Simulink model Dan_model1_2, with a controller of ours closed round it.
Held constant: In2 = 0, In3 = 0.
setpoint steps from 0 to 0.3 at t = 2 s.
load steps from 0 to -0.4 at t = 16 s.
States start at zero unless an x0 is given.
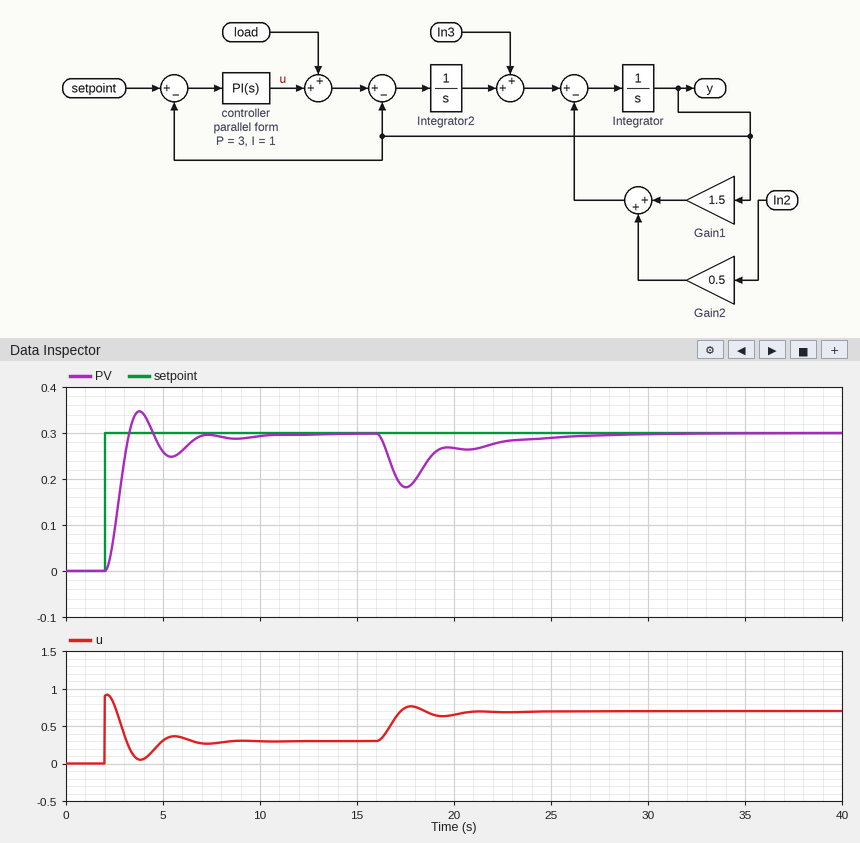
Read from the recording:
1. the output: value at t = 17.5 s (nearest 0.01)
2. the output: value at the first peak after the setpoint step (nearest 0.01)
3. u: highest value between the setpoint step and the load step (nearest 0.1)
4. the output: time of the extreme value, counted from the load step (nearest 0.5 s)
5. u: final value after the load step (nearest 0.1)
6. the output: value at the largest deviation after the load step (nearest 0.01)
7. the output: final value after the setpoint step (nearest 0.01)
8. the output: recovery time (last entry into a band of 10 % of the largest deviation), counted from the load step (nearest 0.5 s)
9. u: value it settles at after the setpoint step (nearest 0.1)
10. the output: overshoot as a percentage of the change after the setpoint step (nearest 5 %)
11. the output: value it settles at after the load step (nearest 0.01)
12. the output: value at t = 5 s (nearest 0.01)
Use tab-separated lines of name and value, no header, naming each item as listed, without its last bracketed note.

the output: value at t = 17.5 s	0.18
the output: value at the first peak after the setpoint step	0.35
u: highest value between the setpoint step and the load step	0.9
the output: time of the extreme value, counted from the load step	1.5 s
u: final value after the load step	0.7
the output: value at the largest deviation after the load step	0.18
the output: final value after the setpoint step	0.30
the output: recovery time (last entry into a band of 10 % of the largest deviation), counted from the load step	8.5 s
u: value it settles at after the setpoint step	0.3
the output: overshoot as a percentage of the change after the setpoint step	15 %
the output: value it settles at after the load step	0.30
the output: value at t = 5 s	0.26
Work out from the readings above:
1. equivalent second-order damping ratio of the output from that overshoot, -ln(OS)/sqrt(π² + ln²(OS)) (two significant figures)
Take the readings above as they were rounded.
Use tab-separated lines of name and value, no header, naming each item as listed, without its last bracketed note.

equivalent second-order damping ratio of the output from that overshoot, -ln(OS)/sqrt(π² + ln²(OS))	0.52
